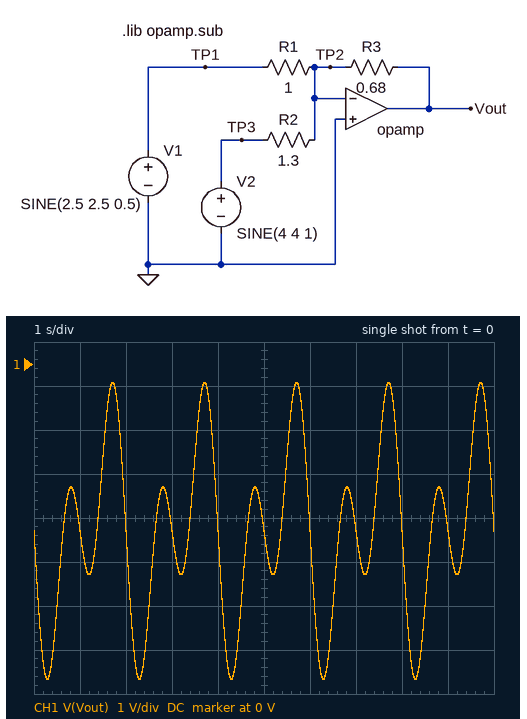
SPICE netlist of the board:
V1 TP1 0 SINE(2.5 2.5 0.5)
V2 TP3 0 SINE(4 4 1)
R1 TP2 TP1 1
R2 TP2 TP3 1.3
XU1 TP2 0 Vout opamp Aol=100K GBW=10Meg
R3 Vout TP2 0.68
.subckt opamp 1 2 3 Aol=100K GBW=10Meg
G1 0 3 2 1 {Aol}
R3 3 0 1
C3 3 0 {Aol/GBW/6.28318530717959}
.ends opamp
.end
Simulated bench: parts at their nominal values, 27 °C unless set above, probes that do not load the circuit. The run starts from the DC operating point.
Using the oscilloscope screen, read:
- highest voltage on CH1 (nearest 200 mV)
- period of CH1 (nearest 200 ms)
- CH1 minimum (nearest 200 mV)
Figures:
-400 mV
2.0 s
-7.2 V
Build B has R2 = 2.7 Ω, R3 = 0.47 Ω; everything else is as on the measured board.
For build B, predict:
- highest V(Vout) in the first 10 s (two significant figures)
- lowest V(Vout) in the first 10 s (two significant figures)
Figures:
-250 mV
-3.5 V
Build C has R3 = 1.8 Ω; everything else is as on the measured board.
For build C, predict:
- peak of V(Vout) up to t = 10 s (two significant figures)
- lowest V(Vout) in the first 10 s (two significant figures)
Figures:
-1.1 V
-19 V
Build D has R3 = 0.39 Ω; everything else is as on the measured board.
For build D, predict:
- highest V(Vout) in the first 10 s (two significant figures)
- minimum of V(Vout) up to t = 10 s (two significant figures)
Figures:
-240 mV
-4.1 V
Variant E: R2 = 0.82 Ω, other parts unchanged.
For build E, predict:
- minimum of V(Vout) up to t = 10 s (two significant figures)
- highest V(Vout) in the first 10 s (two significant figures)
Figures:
-9.6 V
-450 mV
